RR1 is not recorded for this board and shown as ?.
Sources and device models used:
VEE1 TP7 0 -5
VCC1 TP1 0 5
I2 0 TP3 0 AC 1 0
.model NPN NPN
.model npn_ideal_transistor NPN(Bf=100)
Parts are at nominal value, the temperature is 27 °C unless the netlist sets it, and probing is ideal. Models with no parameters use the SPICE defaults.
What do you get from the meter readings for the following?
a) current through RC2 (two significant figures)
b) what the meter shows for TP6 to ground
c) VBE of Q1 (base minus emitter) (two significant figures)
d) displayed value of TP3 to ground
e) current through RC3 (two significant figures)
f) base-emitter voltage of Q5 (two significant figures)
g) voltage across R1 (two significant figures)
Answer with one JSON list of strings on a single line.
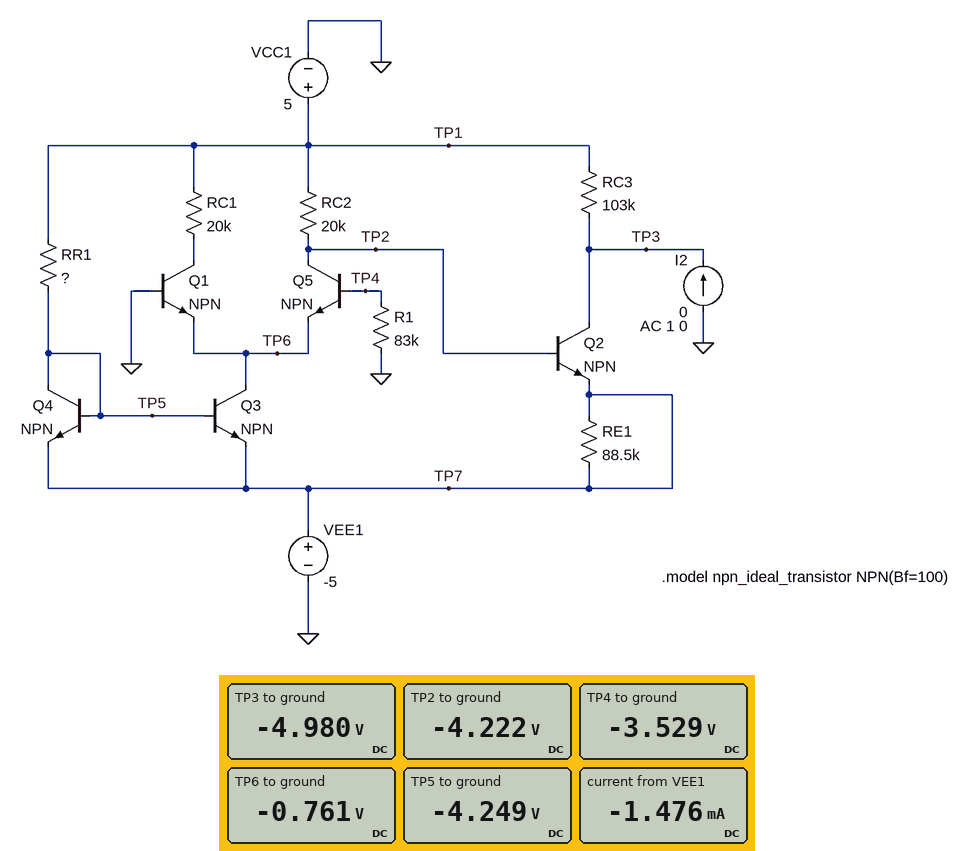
["460 µA", "-0.761 V", "760 mV", "-4.980 V", "97 µA", "-2.8 V", "3.5 V"]
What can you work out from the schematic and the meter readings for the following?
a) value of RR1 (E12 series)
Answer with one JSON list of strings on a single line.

["22 kΩ"]
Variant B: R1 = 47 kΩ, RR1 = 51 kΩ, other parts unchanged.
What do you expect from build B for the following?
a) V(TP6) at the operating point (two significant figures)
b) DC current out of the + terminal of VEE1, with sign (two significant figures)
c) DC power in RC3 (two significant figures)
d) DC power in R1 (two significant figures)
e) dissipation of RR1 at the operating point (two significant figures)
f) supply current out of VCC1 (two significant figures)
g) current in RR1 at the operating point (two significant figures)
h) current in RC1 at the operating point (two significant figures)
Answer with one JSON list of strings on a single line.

["-740 mV", "-1.1 mA", "970 µW", "260 µW", "1.7 mW", "990 µA", "180 µA", "250 µA"]
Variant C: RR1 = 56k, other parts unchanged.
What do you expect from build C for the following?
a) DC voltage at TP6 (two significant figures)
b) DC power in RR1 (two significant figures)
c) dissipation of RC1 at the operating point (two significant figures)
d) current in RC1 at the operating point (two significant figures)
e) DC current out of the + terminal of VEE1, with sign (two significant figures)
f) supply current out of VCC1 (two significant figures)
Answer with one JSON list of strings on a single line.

["-730 mV", "1.5 mW", "820 µW", "200 µA", "-970 µA", "930 µA"]
